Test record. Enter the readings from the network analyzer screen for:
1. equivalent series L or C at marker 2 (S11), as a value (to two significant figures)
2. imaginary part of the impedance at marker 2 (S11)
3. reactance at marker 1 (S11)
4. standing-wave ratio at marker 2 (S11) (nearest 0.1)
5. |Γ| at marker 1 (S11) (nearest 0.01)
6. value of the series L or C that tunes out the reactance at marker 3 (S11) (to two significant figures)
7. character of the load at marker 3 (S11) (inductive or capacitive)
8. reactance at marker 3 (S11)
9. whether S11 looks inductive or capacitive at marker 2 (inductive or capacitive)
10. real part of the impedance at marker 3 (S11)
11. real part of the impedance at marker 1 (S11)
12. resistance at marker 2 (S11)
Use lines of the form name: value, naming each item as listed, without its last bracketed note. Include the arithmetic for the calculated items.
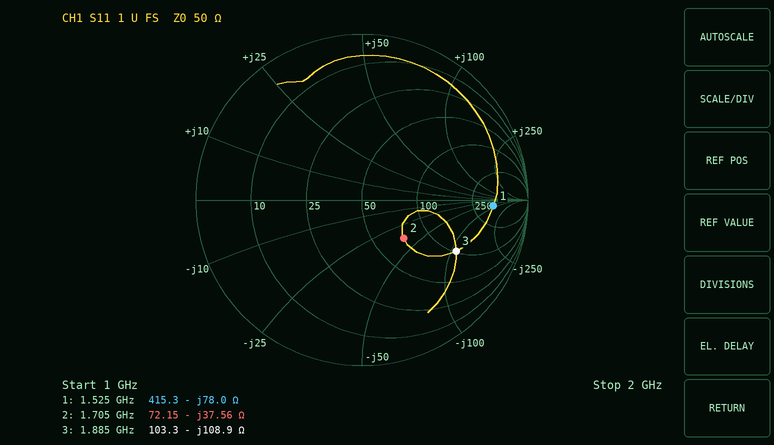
equivalent series L or C at marker 2 (S11), as a value: C = 1/(2π × 1.705 GHz × 37.56 Ω) ≈ 2.5 pF
imaginary part of the impedance at marker 2: -37.56 Ω
reactance at marker 1: -78.0 Ω
standing-wave ratio at marker 2 (S11): 2.0
|Γ| at marker 1 (S11): 0.79
value of the series L or C that tunes out the reactance at marker 3 (S11): L = 108.9 Ω/(2π × 1.885 GHz) ≈ 9.2 nH
character of the load at marker 3 (S11): capacitive
reactance at marker 3: -108.9 Ω
whether S11 looks inductive or capacitive at marker 2: capacitive
real part of the impedance at marker 3: 103.3 Ω
real part of the impedance at marker 1: 415.3 Ω
resistance at marker 2: 72.15 Ω
